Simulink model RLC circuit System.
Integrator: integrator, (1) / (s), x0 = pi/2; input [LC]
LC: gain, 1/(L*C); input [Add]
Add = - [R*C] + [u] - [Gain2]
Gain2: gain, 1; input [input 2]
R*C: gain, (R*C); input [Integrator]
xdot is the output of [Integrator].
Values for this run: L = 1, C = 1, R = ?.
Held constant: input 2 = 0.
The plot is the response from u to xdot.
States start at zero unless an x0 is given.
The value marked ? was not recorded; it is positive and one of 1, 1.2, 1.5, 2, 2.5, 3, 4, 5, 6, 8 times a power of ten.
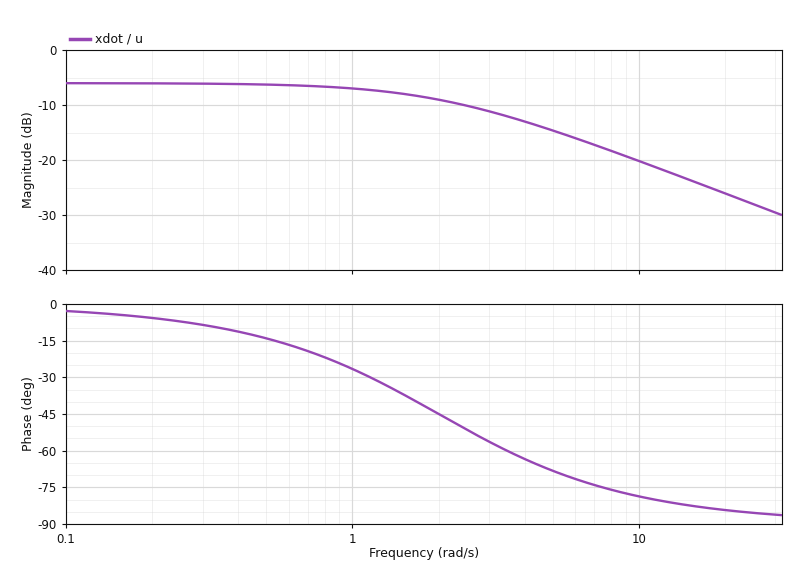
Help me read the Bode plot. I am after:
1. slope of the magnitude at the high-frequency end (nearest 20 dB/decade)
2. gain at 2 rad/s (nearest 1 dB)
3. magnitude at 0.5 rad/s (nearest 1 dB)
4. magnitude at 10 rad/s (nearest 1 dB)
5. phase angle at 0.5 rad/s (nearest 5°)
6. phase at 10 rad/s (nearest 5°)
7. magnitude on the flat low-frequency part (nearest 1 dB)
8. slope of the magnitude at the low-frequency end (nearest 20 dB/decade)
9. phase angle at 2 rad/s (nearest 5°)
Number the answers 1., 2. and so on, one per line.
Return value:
1. -20 dB/decade
2. -9 dB
3. -6 dB
4. -20 dB
5. -15°
6. -80°
7. -6 dB
8. 0 dB/decade
9. -45°
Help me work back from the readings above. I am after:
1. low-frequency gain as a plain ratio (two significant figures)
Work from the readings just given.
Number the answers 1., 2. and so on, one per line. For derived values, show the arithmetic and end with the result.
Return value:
1. 10^(-6 / 20) = 0.50
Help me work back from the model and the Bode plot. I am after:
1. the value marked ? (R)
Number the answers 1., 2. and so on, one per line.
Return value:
1. 2
